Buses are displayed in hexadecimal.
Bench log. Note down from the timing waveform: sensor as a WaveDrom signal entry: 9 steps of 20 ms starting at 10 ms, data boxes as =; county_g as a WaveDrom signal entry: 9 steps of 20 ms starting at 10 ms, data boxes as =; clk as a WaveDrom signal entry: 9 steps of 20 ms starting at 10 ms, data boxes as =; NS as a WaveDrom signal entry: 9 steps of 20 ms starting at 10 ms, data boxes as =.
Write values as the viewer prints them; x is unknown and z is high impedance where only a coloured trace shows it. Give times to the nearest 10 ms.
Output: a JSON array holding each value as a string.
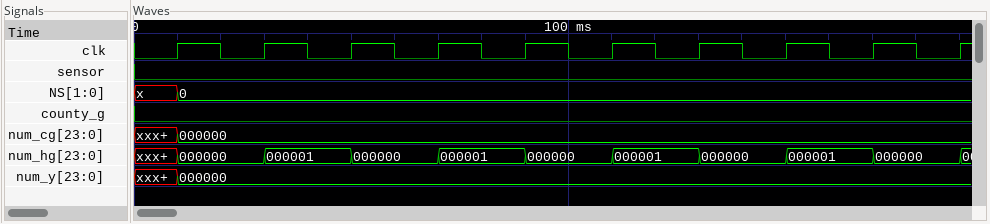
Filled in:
["{name: 'sensor', wave: '0........'}", "{name: 'county_g', wave: '0........'}", "{name: 'clk', wave: 'p........'}", "{name: 'NS', wave: '=........', data: '0'}"]
